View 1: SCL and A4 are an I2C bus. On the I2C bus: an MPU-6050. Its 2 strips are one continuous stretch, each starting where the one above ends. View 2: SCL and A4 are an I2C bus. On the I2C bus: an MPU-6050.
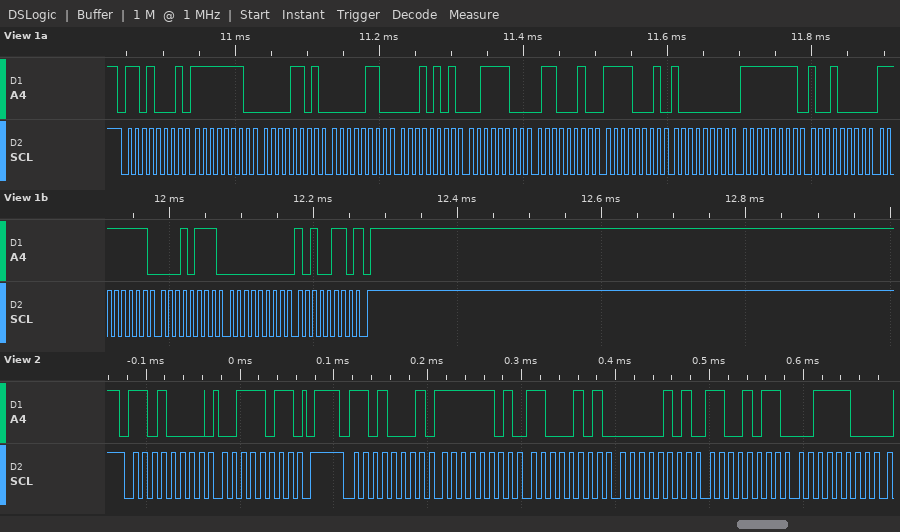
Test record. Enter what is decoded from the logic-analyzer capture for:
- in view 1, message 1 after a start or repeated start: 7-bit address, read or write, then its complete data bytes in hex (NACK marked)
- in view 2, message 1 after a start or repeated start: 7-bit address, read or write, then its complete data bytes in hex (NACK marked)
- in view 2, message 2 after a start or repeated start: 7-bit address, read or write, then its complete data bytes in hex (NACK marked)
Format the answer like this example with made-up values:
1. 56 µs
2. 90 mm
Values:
1. 0x68 read: FE 0D 06 15 3C 62 F1 80 FF 90 FF 17 00 A6 NACK
2. 0x68 write: 3B
3. 0x68 read: FD C5 05 CB 3C
